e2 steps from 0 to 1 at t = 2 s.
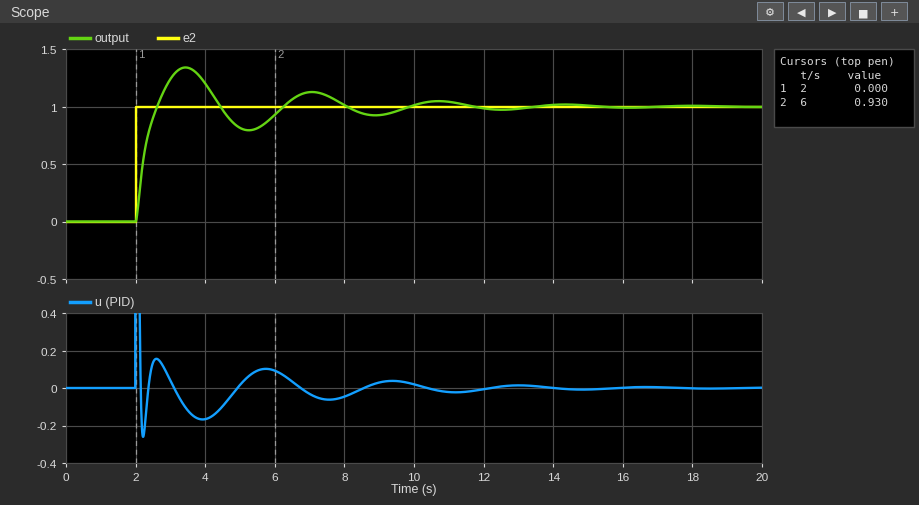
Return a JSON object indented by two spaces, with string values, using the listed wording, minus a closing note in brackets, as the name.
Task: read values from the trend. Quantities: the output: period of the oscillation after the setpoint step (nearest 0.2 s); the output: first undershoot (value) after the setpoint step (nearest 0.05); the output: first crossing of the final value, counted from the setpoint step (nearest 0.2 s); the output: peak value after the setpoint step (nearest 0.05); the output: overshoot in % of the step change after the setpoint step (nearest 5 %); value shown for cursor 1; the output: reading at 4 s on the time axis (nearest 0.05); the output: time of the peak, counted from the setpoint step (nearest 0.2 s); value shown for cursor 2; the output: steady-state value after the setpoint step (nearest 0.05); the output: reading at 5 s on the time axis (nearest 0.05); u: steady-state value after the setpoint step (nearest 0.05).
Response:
{
  "the output: period of the oscillation after the setpoint step": "3.6 s",
  "the output: first undershoot (value) after the setpoint step": "0.80",
  "the output: first crossing of the final value, counted from the setpoint step": "0.6 s",
  "the output: peak value after the setpoint step": "1.35",
  "the output: overshoot in % of the step change after the setpoint step": "35 %",
  "value shown for cursor 1": "0.000",
  "the output: reading at 4 s on the time axis": "1.20",
  "the output: time of the peak, counted from the setpoint step": "1.4 s",
  "value shown for cursor 2": "0.930",
  "the output: steady-state value after the setpoint step": "1.00",
  "the output: reading at 5 s on the time axis": "0.80",
  "u: steady-state value after the setpoint step": "0.00"
}
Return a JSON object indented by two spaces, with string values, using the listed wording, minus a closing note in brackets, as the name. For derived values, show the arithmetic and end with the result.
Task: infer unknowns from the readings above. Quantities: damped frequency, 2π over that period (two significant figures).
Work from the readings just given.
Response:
{
  "damped frequency, 2π over that period": "2π / 3.6 = 1.7 rad/s"
}
